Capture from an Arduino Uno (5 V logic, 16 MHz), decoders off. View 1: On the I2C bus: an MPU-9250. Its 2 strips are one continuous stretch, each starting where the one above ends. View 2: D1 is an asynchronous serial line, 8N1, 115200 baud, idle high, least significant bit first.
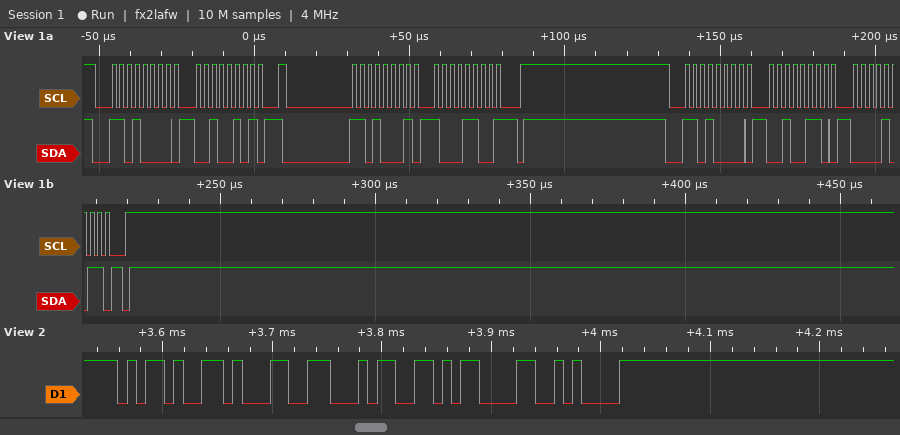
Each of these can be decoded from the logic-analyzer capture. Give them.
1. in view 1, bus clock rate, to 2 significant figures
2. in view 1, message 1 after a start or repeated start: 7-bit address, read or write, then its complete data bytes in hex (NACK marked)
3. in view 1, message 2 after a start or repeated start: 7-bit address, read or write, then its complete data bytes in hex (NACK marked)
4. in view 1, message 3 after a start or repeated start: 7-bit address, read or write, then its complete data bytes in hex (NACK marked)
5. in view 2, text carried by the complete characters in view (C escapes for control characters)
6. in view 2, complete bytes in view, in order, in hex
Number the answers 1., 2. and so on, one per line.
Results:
1. 400 kHz
2. 0x68 write: 25
3. 0x68 read: 8C NACK
4. 0x68 write: 26 0B
5. "-14\r\n"
6. 2D 31 34 0D 0A
